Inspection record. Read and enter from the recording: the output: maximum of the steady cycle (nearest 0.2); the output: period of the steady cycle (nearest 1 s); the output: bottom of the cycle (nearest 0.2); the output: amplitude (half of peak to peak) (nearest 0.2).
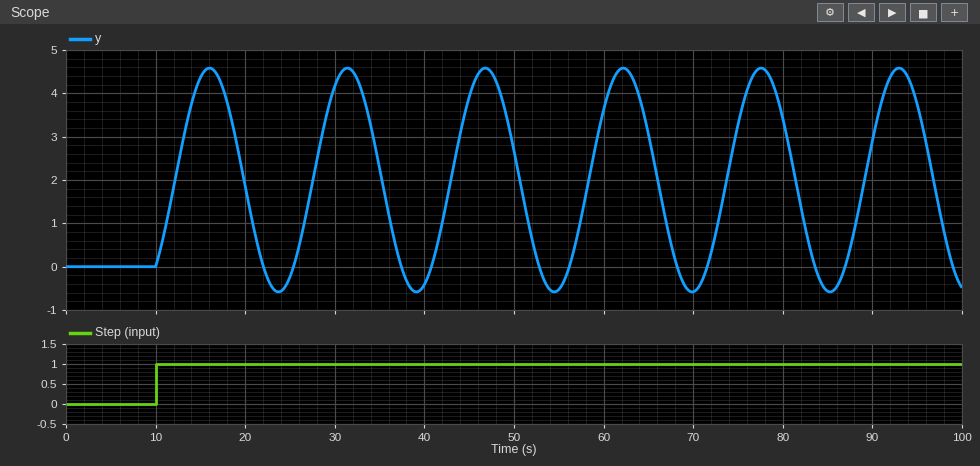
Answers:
4.6
15 s
-0.6
2.6
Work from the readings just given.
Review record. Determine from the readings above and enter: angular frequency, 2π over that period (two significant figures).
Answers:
0.42 rad/s
